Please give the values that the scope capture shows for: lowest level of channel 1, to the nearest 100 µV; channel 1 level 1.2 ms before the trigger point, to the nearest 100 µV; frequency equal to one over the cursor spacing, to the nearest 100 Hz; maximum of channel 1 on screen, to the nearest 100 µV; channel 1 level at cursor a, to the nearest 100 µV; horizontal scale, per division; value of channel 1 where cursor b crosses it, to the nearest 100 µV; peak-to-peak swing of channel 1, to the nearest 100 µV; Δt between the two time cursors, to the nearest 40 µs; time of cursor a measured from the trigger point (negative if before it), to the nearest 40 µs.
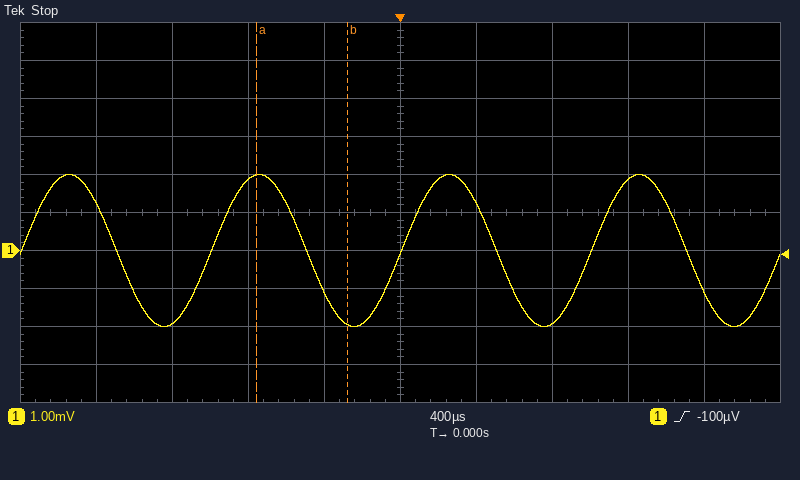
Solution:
-2.0 mV
-1.9 mV
2.1 kHz
2.0 mV
2.0 mV
400 µs
-1.9 mV
4.0 mV
480 µs
-760 µs
